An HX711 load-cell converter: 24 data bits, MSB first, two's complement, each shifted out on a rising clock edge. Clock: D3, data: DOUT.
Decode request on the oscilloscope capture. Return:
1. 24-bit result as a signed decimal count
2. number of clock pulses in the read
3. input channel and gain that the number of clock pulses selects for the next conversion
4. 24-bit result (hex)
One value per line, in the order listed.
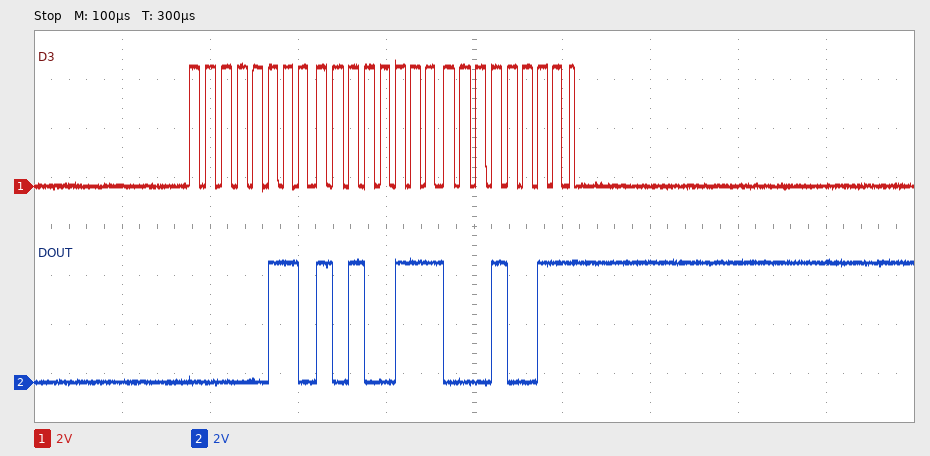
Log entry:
435987
25
channel A, gain 128
0x06A713
